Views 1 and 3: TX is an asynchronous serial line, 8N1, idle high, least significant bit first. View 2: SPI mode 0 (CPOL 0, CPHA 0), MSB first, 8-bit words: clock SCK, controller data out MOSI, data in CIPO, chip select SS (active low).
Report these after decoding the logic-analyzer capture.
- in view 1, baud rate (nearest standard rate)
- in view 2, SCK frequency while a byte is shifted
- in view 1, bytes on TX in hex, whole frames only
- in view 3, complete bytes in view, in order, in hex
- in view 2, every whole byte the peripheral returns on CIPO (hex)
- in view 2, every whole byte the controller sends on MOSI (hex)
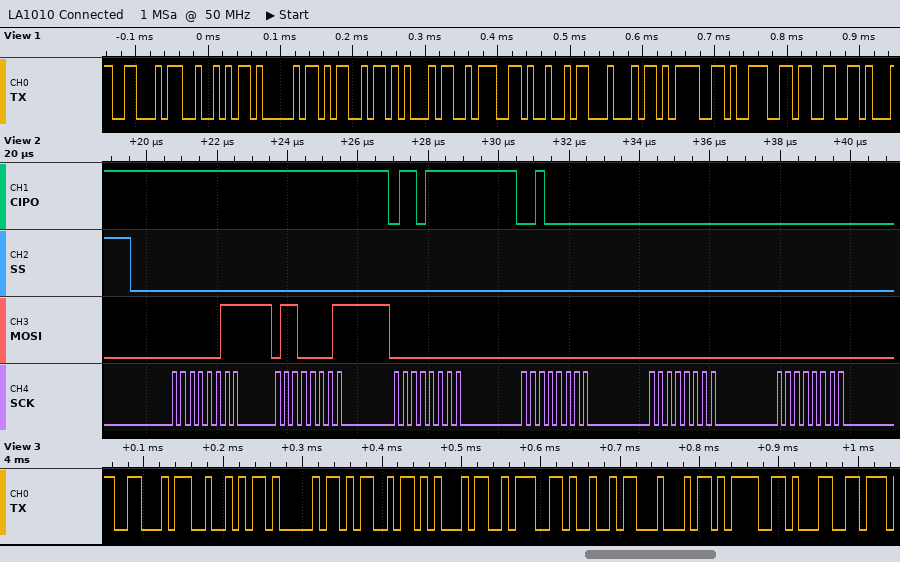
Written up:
115200 baud
4 MHz
46 52 41 4D 45 3A 49 44 3D 39 33
46 52 41 4D 45 3A 49 44 3D 31
0xFF 0xFF 0x6F 0x20 0x00 0x00
0x03 0x61 0x00 0x00 0x00 0x00
